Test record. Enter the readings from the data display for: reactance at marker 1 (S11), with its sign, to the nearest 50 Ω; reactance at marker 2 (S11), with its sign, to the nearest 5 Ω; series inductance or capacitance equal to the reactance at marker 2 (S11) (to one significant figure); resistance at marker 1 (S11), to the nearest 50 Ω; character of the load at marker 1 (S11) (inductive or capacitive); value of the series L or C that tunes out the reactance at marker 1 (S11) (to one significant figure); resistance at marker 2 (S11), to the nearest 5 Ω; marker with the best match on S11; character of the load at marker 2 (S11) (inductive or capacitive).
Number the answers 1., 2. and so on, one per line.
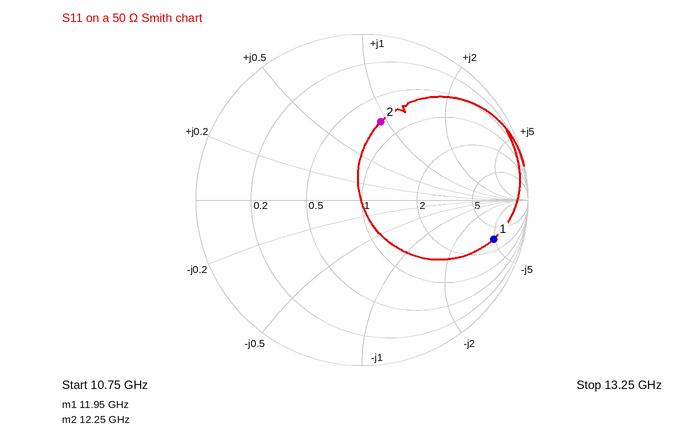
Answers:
1. -250 Ω
2. +45 Ω
3. 600 pH
4. 150 Ω
5. capacitive
6. 3 nH
7. 40 Ω
8. marker 2
9. inductive
